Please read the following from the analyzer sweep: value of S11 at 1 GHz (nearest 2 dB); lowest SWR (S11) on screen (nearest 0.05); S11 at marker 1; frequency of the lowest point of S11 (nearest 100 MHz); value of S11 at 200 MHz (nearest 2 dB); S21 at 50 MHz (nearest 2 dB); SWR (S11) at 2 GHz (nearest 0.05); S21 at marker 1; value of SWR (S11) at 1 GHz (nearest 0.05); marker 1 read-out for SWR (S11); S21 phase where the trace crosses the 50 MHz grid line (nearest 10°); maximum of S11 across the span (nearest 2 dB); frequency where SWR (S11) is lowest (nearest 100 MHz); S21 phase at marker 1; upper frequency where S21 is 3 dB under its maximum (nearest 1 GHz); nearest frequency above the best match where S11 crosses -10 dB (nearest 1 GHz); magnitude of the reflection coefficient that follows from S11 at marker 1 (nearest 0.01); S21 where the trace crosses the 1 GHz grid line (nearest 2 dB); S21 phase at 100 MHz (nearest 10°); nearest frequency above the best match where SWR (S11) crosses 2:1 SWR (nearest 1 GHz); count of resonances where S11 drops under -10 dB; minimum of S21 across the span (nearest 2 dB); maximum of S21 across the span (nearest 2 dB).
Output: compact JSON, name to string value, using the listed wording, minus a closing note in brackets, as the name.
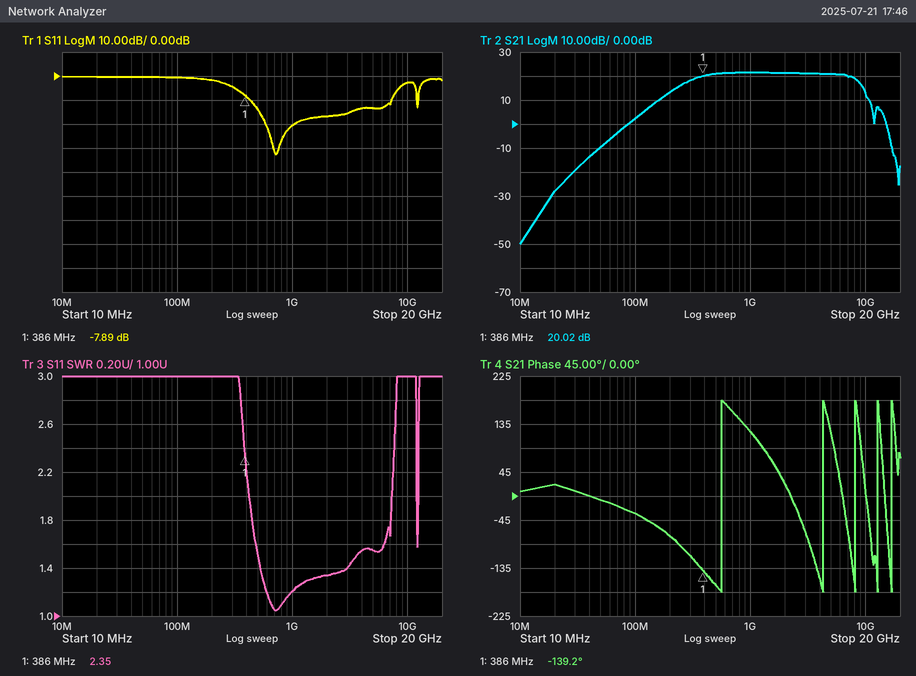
{"value of S11 at 1 GHz": "-20 dB", "lowest SWR (S11) on screen": "1.05", "S11 at marker 1": "-7.89 dB", "frequency of the lowest point of S11": "700 MHz", "value of S11 at 200 MHz": "-2 dB", "S21 at 50 MHz": "-10 dB", "SWR (S11) at 2 GHz": "1.35", "S21 at marker 1": "20.02 dB", "value of SWR (S11) at 1 GHz": "1.20", "marker 1 read-out for SWR": "2.35", "S21 phase where the trace crosses the 50 MHz grid line": "-10°", "maximum of S11 across the span": "0 dB", "frequency where SWR (S11) is lowest": "700 MHz", "S21 phase at marker 1": "-139.2°", "upper frequency where S21 is 3 dB under its maximum": "8 GHz", "nearest frequency above the best match where S11 crosses -10 dB": "7 GHz", "magnitude of the reflection coefficient that follows from S11 at marker 1": "0.40", "S21 where the trace crosses the 1 GHz grid line": "22 dB", "S21 phase at 100 MHz": "-30°", "nearest frequency above the best match where SWR (S11) crosses 2:1 SWR": "7 GHz", "count of resonances where S11 drops under -10 dB": "2", "minimum of S21 across the span": "-50 dB", "maximum of S21 across the span": "22 dB"}
